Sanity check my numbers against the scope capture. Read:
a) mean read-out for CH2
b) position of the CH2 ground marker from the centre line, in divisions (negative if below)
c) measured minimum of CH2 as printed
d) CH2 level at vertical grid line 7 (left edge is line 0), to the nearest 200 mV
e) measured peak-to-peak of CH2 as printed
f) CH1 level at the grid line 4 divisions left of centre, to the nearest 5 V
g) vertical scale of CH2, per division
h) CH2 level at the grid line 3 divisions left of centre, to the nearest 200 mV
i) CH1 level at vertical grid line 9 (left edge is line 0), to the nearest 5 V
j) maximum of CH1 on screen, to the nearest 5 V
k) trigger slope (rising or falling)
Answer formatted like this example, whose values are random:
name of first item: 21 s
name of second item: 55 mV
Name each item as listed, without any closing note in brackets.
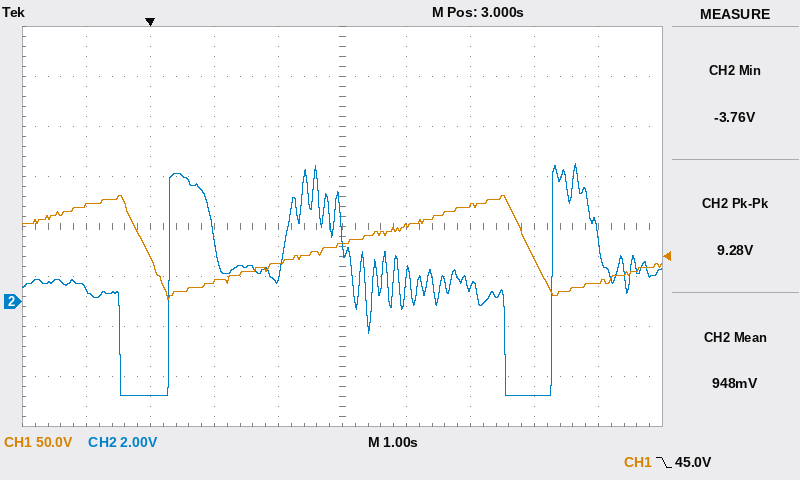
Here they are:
mean read-out for CH2: 948 mV
position of the CH2 ground marker from the centre line, in divisions: -1.5 div
measured minimum of CH2 as printed: -3.76 V
CH2 level at vertical grid line 7 (left edge is line 0), to the nearest 200 mV: 600 mV
measured peak-to-peak of CH2 as printed: 9.28 V
CH1 level at the grid line 4 divisions left of centre, to the nearest 5 V: 95 V
vertical scale of CH2, per division: 2 V
CH2 level at the grid line 3 divisions left of centre, to the nearest 200 mV: -3.8 V
CH1 level at vertical grid line 9 (left edge is line 0), to the nearest 5 V: 20 V
maximum of CH1 on screen, to the nearest 5 V: 105 V
trigger slope: falling
